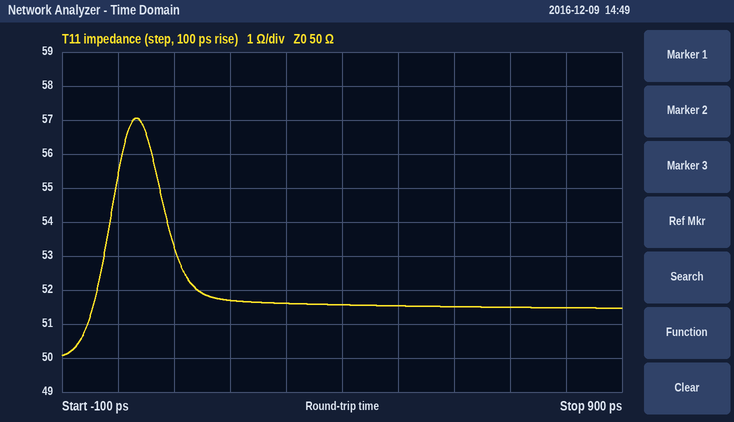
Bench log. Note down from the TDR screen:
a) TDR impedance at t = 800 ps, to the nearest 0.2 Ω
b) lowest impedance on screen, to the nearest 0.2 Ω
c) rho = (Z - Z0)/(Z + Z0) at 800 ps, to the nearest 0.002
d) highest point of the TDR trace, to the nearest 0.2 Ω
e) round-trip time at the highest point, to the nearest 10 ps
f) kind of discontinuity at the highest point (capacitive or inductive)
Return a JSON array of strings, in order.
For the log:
["51.4 Ω", "50.0 Ω", "+0.014", "57.0 Ω", "30 ps", "inductive"]
